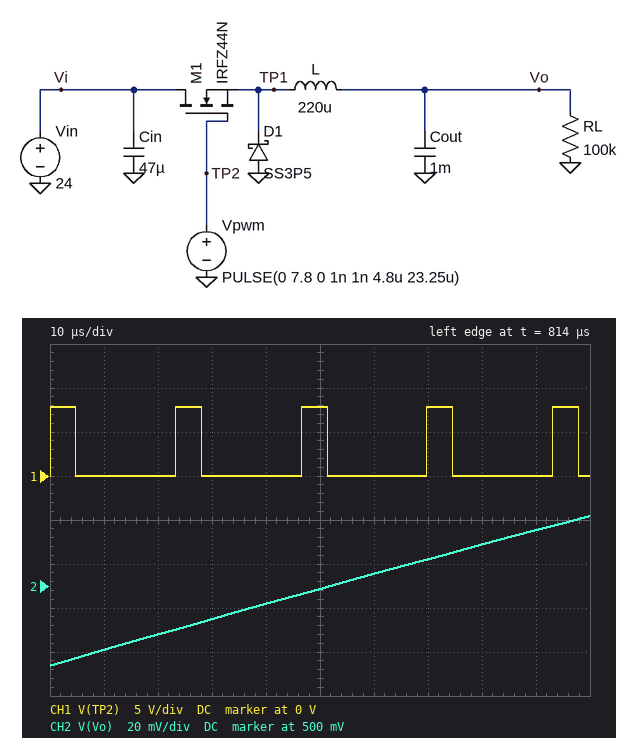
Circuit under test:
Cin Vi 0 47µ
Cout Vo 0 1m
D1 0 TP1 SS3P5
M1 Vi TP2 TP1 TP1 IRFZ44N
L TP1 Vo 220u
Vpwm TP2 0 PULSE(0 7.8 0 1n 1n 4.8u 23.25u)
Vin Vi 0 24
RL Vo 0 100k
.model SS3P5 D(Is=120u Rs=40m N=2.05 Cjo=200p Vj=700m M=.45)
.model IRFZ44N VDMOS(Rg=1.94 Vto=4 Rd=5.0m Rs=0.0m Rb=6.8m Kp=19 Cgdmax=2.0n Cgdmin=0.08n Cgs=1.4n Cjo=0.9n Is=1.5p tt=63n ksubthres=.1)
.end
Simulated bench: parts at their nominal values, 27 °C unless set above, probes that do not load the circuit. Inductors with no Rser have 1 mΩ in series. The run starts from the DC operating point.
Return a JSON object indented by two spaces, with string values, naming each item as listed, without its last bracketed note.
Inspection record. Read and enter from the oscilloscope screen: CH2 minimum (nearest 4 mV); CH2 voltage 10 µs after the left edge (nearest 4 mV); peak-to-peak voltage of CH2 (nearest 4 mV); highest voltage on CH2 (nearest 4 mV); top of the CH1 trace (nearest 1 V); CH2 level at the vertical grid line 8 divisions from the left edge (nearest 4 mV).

{
  "CH2 minimum": "464 mV",
  "CH2 voltage 10 µs after the left edge": "472 mV",
  "peak-to-peak voltage of CH2": "68 mV",
  "highest voltage on CH2": "532 mV",
  "top of the CH1 trace": "8 V",
  "CH2 level at the vertical grid line 8 divisions from the left edge": "520 mV"
}
